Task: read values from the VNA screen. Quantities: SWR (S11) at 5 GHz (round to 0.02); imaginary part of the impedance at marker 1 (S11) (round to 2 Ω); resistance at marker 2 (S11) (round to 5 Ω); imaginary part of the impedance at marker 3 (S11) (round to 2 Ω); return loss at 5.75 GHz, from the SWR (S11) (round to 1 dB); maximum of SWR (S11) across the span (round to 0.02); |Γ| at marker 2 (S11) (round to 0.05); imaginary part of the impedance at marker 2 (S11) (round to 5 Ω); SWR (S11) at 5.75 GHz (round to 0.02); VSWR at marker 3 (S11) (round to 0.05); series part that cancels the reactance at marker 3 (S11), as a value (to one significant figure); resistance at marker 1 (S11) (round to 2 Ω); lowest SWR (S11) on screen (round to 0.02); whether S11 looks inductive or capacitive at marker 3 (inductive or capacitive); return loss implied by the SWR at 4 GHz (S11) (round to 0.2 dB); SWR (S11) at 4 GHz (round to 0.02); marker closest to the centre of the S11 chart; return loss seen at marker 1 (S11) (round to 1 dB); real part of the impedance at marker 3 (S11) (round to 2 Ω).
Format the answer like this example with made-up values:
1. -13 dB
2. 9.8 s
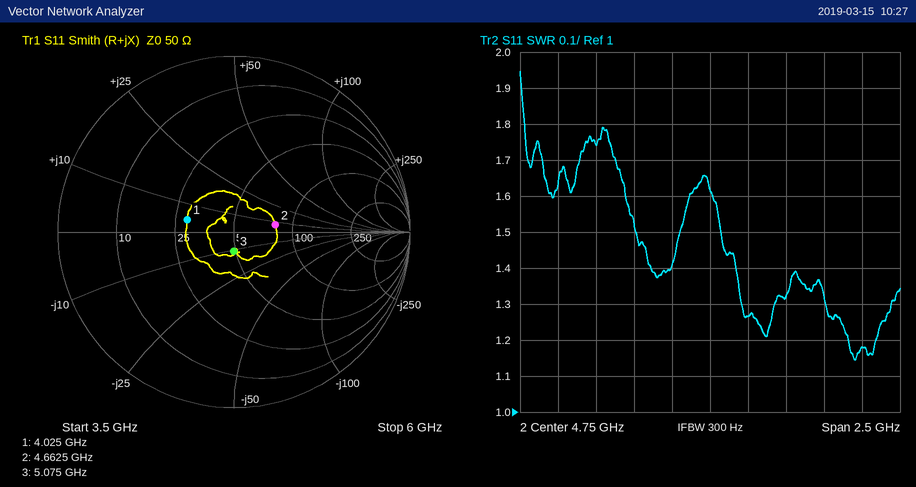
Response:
1. 1.26
2. +4 Ω
3. 80 Ω
4. -10 Ω
5. 22 dB
6. 1.94
7. 0.25
8. +5 Ω
9. 1.18
10. 1.25
11. 300 pH
12. 28 Ω
13. 1.14
14. capacitive
15. 11.4 dB
16. 1.74
17. marker 3
18. 11 dB
19. 48 Ω
